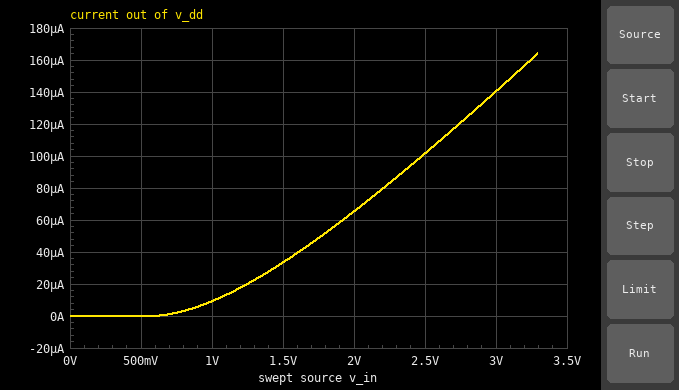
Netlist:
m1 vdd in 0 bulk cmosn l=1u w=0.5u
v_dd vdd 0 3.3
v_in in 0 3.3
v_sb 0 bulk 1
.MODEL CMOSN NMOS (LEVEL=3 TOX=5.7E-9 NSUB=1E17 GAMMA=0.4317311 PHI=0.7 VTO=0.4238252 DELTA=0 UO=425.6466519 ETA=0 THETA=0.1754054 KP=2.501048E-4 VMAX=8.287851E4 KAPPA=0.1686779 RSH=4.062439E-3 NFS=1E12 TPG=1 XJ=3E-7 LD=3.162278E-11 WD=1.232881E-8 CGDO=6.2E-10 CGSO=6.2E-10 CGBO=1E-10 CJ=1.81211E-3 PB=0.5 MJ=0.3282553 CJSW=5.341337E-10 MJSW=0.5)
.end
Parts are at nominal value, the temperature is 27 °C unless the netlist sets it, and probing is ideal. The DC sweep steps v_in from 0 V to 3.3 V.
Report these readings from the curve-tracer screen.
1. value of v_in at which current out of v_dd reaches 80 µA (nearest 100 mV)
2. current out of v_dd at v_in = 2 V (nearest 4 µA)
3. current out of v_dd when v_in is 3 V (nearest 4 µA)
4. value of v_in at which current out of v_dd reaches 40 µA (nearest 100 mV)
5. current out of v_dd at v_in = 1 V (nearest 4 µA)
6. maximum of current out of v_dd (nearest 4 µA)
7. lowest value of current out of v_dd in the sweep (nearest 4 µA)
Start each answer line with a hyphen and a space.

- 2.2 V
- 64 µA
- 140 µA
- 1.6 V
- 8 µA
- 164 µA
- 0 A
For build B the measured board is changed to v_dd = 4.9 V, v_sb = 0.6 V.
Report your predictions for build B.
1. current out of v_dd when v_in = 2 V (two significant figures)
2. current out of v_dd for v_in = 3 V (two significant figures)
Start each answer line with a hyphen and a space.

- 70 µA
- 150 µA
